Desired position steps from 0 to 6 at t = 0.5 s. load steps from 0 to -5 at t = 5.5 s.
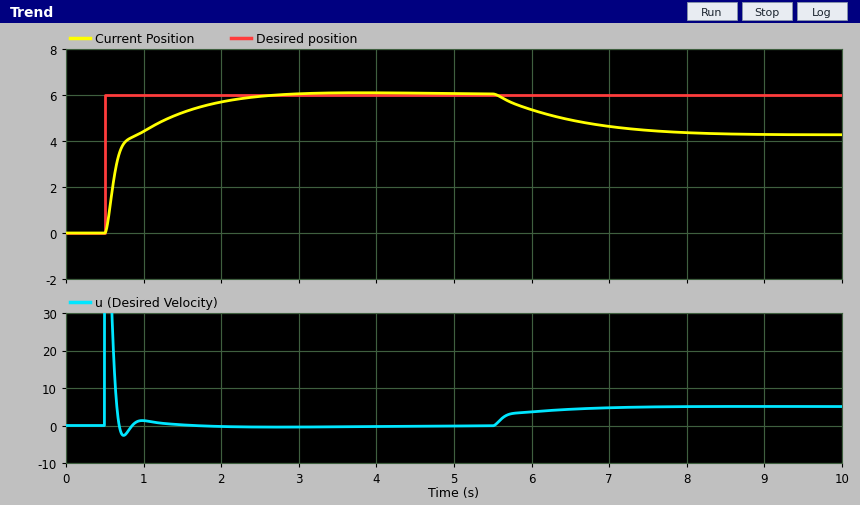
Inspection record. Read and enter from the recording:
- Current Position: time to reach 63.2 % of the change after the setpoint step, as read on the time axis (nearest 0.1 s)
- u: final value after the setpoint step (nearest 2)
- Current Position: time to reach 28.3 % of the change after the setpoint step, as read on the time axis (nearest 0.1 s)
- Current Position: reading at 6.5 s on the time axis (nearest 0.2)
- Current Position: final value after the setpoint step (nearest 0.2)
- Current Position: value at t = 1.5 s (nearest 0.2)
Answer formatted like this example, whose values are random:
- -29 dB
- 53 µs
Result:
- 0.7 s
- 0
- 0.6 s
- 5.0
- 6.0
- 5.2
